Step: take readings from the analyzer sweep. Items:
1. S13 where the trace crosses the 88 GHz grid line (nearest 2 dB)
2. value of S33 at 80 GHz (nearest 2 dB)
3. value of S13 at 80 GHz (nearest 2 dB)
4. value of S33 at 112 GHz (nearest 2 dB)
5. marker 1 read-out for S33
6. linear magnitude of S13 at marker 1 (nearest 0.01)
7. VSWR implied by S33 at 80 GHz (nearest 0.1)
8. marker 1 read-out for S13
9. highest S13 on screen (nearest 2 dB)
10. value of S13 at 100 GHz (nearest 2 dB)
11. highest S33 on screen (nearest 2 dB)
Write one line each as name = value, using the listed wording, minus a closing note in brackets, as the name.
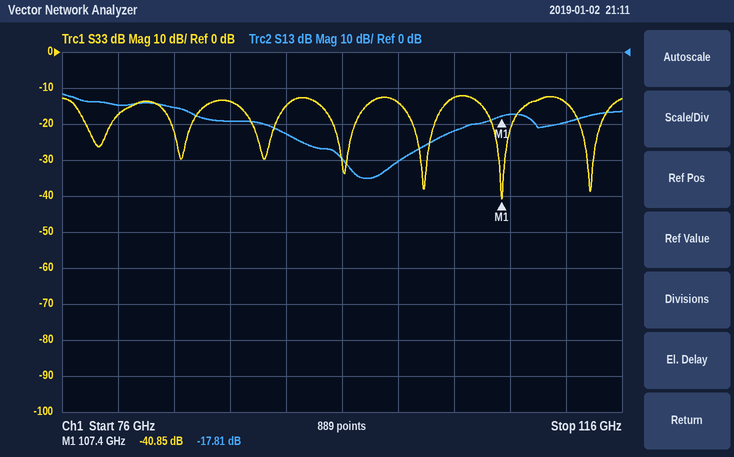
S13 where the trace crosses the 88 GHz grid line = -20 dB
value of S33 at 80 GHz = -18 dB
value of S13 at 80 GHz = -14 dB
value of S33 at 112 GHz = -14 dB
marker 1 read-out for S33 = -40.85 dB
linear magnitude of S13 at marker 1 = 0.13
VSWR implied by S33 at 80 GHz = 1.3
marker 1 read-out for S13 = -17.81 dB
highest S13 on screen = -12 dB
value of S13 at 100 GHz = -30 dB
highest S33 on screen = -12 dB
